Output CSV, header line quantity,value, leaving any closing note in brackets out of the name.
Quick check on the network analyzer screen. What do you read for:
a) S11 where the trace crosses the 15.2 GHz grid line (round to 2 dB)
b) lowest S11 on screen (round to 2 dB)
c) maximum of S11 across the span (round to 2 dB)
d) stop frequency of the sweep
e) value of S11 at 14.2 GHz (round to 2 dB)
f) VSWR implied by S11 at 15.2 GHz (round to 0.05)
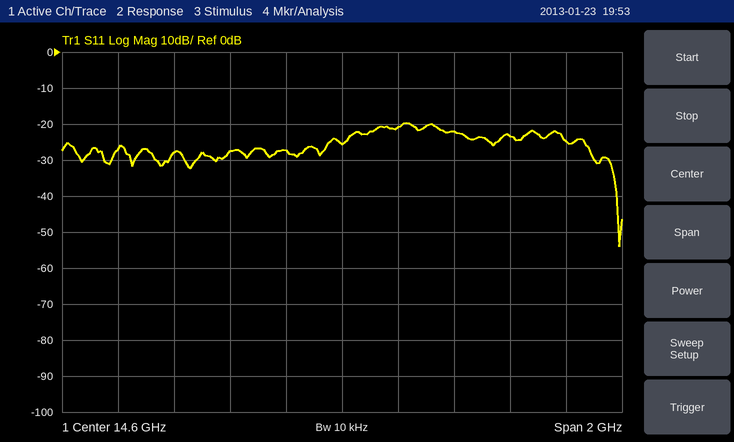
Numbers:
quantity,value
S11 where the trace crosses the 15.2 GHz grid line,-24 dB
lowest S11 on screen,-54 dB
maximum of S11 across the span,-20 dB
stop frequency of the sweep,15.6 GHz
value of S11 at 14.2 GHz,-28 dB
VSWR implied by S11 at 15.2 GHz,1.15
